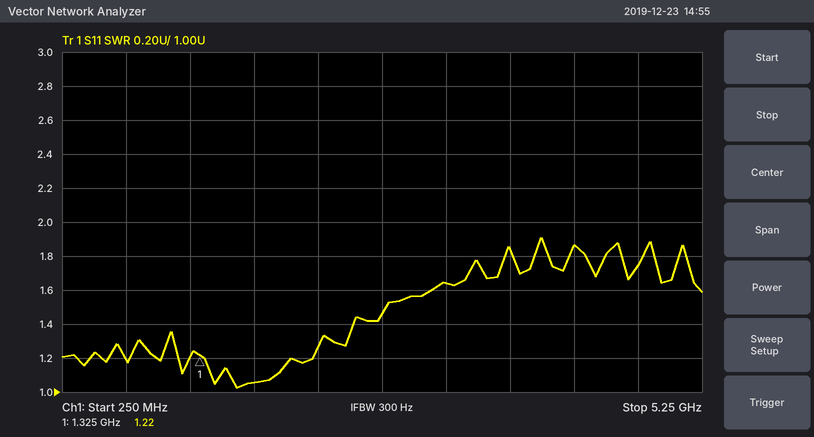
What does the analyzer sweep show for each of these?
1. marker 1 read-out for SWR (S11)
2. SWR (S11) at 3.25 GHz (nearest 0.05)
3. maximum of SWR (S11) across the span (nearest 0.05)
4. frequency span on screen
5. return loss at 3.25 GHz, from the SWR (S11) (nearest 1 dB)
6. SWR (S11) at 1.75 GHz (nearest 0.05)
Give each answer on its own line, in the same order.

1.22
1.65
1.90
5 GHz
12 dB
1.05
